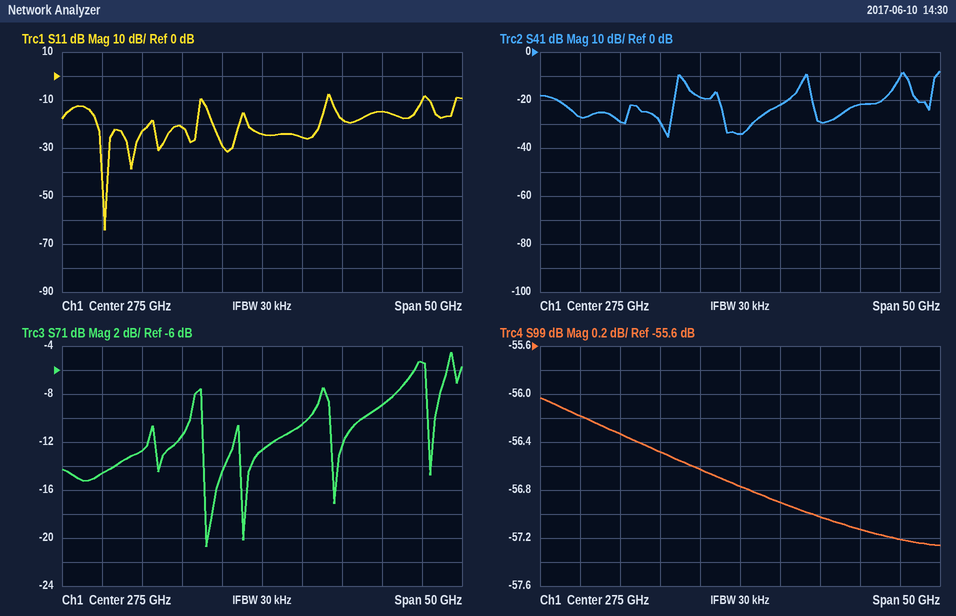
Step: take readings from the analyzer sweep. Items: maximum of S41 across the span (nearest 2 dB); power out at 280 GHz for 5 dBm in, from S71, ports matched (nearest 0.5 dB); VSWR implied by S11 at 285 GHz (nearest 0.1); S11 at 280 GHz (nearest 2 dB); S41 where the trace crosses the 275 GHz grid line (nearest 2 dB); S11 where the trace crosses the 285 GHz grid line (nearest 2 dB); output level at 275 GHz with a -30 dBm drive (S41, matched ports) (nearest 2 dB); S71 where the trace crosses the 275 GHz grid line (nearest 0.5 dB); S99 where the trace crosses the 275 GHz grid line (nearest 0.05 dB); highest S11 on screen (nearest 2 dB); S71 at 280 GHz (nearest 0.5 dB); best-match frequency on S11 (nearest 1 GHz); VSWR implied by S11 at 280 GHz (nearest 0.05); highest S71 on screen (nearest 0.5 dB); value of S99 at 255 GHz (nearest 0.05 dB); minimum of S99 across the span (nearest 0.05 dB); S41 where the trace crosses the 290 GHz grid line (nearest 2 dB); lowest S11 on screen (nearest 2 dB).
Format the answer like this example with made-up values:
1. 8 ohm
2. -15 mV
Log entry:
1. -8 dB
2. -5.5 dBm
3. 1.3
4. -26 dB
5. -34 dB
6. -18 dB
7. -64 dBm
8. -12.5 dB
9. -56.75 dB
10. -8 dB
11. -10.5 dB
12. 255 GHz
13. 1.10
14. -4.5 dB
15. -56.20 dB
16. -57.25 dB
17. -22 dB
18. -64 dB
